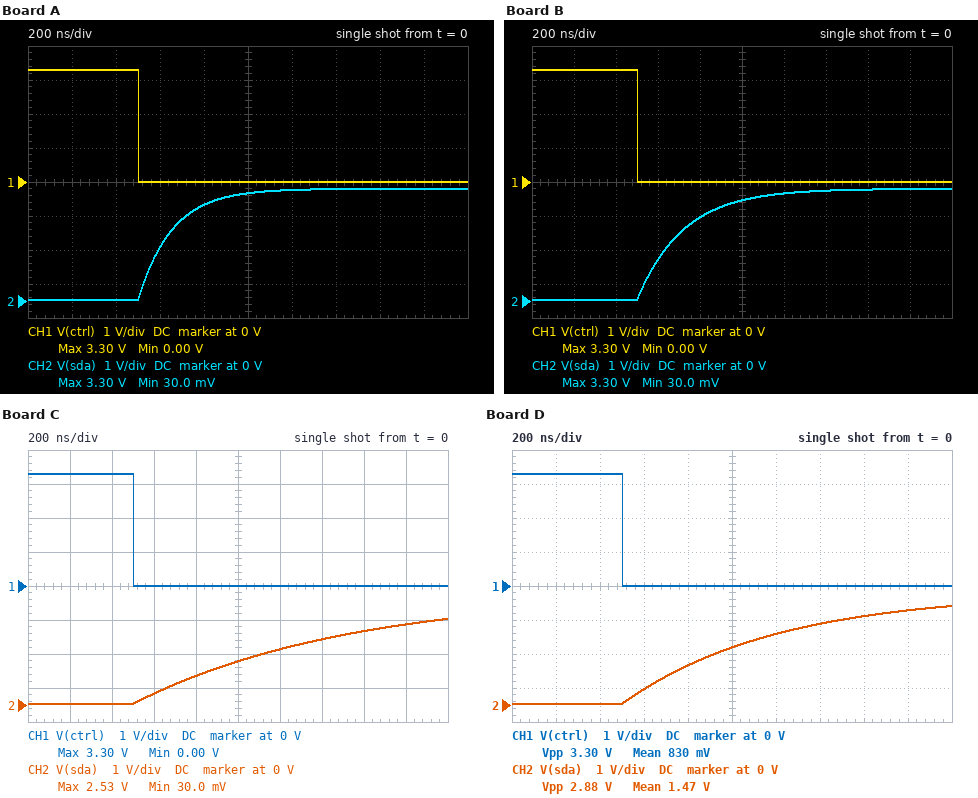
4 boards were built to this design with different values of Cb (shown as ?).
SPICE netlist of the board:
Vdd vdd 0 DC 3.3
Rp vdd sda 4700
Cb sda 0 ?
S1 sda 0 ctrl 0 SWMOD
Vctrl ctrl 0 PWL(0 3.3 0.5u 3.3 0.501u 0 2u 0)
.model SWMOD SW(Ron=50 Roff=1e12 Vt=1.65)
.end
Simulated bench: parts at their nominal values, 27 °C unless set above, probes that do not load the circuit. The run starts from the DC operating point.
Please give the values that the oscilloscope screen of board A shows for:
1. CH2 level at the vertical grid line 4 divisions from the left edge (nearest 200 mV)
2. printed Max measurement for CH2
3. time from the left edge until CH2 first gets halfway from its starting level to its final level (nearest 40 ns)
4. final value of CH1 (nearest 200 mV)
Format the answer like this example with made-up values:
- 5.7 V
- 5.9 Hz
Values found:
- 2.8 V
- 3.30 V
- 600 ns
- 0 V
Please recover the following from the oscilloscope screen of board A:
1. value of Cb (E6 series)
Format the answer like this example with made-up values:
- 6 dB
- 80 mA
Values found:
- 33 pF
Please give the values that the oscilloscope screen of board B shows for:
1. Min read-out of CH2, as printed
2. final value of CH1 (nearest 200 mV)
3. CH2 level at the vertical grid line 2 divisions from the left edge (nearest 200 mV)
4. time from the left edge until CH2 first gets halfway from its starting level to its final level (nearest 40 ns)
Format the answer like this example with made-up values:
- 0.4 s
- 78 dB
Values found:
- 30.0 mV
- 0 V
- 0 V
- 640 ns
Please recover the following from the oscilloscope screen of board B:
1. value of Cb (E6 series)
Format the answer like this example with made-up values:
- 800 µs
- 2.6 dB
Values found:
- 47 pF
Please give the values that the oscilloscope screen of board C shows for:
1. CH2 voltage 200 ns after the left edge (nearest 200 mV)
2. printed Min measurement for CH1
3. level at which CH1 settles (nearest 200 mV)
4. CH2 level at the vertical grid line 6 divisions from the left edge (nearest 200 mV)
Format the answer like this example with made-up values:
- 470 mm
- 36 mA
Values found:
- 0 V
- 0.00 V
- 0 V
- 1.6 V
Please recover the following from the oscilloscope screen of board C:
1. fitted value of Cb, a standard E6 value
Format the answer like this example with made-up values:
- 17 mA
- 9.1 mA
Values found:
- 220 pF
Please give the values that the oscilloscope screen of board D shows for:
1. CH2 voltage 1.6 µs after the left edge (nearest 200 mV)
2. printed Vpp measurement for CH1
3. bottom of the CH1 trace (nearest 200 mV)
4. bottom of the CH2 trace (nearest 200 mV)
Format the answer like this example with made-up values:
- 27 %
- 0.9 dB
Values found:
- 2.6 V
- 3.30 V
- 0 V
- 0 V
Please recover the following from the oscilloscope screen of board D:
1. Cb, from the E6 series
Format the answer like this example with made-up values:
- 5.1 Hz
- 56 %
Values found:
- 150 pF
